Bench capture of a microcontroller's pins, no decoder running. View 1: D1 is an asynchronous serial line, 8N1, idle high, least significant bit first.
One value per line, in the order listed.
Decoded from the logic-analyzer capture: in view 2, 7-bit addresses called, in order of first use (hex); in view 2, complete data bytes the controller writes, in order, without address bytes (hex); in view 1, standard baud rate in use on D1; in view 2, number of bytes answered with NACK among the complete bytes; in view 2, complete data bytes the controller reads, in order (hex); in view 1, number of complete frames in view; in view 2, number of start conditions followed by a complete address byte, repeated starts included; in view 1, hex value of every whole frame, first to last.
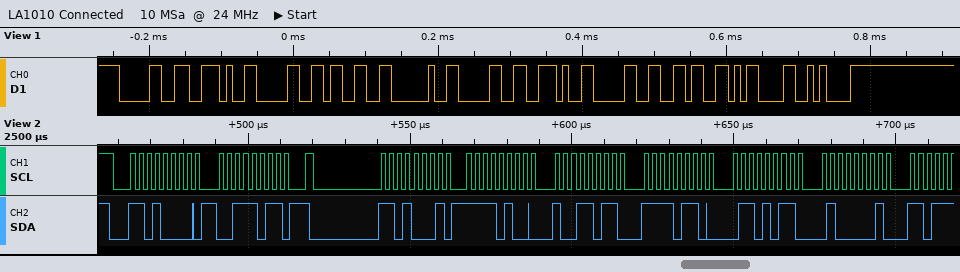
0x68
3B
115200 baud
0
F4 9B F6 6B 41
11
2
0x30 0x2E 0x30 0x33 0x20 0x30 0x2E 0x30 0x36 0x0D 0x0A
